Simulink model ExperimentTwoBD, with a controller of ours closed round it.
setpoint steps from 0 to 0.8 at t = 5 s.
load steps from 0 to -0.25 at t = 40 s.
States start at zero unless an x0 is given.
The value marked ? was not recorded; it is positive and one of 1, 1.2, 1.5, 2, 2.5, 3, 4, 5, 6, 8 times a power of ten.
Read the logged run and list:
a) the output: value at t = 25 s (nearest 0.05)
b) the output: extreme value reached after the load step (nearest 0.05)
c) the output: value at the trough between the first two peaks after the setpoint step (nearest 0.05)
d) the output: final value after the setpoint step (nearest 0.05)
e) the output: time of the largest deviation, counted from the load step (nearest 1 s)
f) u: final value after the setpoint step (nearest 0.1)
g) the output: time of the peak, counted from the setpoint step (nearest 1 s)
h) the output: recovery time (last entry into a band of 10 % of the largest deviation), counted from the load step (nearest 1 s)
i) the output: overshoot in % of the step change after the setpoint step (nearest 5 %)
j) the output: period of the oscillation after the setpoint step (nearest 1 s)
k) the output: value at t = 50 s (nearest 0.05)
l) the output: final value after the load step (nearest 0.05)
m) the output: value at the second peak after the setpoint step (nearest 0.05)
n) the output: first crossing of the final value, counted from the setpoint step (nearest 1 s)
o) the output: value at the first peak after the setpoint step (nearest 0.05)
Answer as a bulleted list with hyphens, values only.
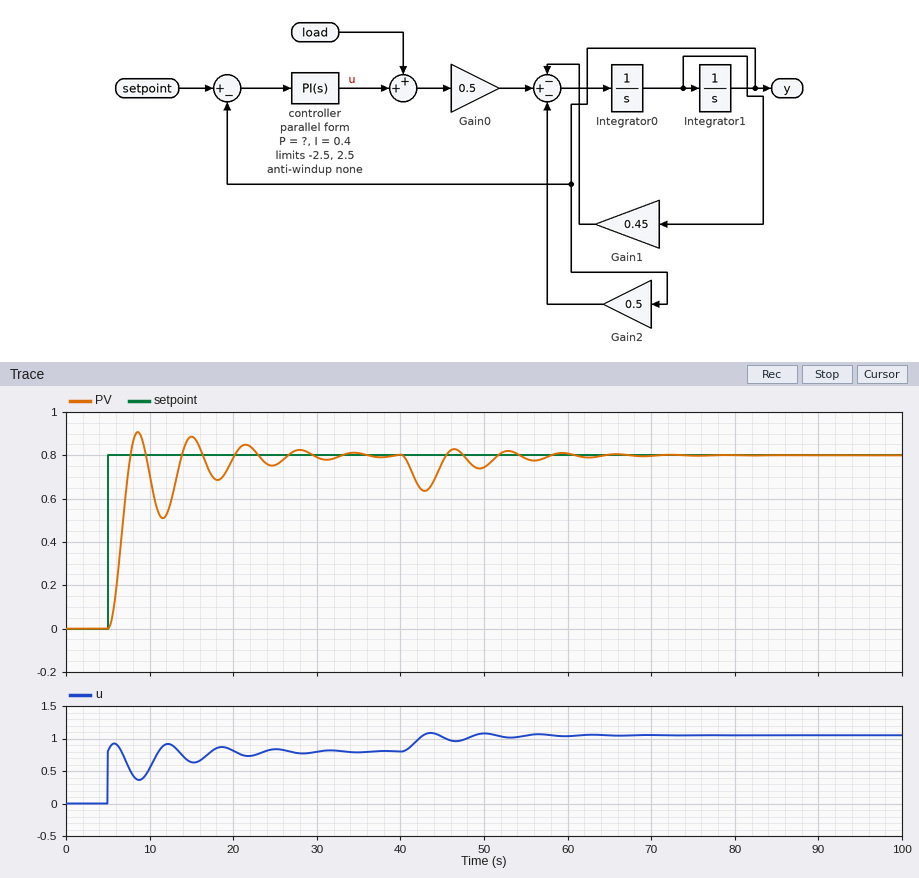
- 0.75
- 0.65
- 0.50
- 0.80
- 3 s
- 0.8
- 4 s
- 17 s
- 15 %
- 6 s
- 0.75
- 0.80
- 0.90
- 3 s
- 0.90
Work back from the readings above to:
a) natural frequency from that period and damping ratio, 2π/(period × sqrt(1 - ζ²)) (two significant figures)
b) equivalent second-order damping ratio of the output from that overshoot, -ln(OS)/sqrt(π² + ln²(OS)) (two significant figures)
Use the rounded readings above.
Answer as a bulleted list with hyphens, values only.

- 1.2 rad/s
- 0.52
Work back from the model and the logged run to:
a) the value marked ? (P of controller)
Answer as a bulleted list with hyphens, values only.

- 1
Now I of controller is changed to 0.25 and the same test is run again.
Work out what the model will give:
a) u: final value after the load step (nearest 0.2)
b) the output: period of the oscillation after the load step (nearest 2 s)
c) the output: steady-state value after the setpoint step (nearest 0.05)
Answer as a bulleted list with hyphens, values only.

- 1.0
- 6 s
- 0.80
